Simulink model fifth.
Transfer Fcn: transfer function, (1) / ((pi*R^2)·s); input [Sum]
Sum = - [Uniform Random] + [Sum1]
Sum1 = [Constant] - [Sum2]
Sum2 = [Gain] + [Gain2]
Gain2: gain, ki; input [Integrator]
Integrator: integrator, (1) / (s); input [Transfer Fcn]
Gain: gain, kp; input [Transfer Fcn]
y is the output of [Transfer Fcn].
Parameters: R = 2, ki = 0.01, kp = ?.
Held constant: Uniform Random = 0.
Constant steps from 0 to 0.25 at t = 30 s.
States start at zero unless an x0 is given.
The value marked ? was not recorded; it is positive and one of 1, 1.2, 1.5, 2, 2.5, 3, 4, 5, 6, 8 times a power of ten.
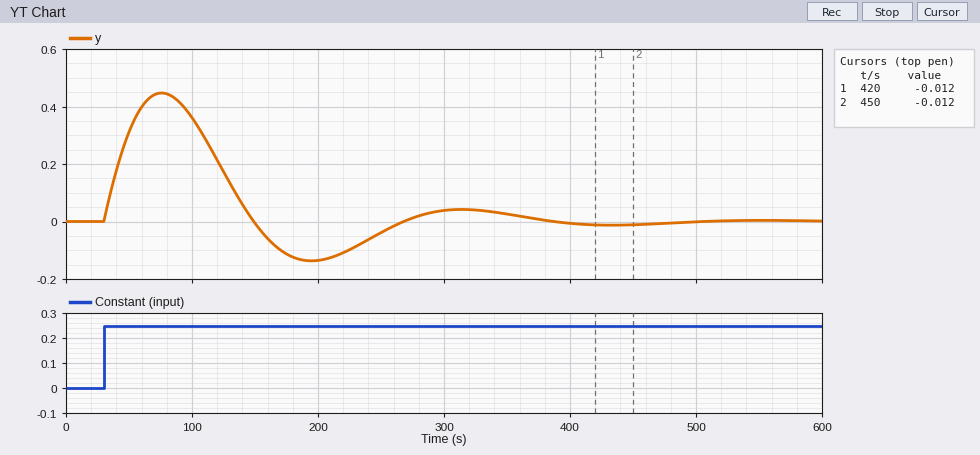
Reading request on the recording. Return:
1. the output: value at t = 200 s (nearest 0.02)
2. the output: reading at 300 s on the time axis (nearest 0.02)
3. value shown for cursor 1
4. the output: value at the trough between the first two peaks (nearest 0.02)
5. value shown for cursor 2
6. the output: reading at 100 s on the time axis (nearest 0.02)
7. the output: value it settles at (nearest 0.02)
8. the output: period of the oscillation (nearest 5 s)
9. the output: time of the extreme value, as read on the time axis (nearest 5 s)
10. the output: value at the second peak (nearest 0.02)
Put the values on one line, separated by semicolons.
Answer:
-0.14; 0.04; -0.012; -0.14; -0.012; 0.36; 0.00; 240 s; 75 s; 0.04
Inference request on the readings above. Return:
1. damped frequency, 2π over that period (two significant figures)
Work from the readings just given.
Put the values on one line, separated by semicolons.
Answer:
0.026 rad/s
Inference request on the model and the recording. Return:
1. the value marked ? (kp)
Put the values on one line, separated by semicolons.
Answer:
0.25
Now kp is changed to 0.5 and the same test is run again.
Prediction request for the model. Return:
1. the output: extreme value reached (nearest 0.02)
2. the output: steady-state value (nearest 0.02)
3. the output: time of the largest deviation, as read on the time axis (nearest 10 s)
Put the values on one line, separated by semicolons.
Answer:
0.32; 0.00; 70 s
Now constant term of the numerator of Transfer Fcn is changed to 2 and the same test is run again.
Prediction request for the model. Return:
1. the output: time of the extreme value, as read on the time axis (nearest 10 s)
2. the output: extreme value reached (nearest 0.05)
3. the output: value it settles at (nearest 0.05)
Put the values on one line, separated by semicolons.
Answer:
60 s; 0.55; 0.00
